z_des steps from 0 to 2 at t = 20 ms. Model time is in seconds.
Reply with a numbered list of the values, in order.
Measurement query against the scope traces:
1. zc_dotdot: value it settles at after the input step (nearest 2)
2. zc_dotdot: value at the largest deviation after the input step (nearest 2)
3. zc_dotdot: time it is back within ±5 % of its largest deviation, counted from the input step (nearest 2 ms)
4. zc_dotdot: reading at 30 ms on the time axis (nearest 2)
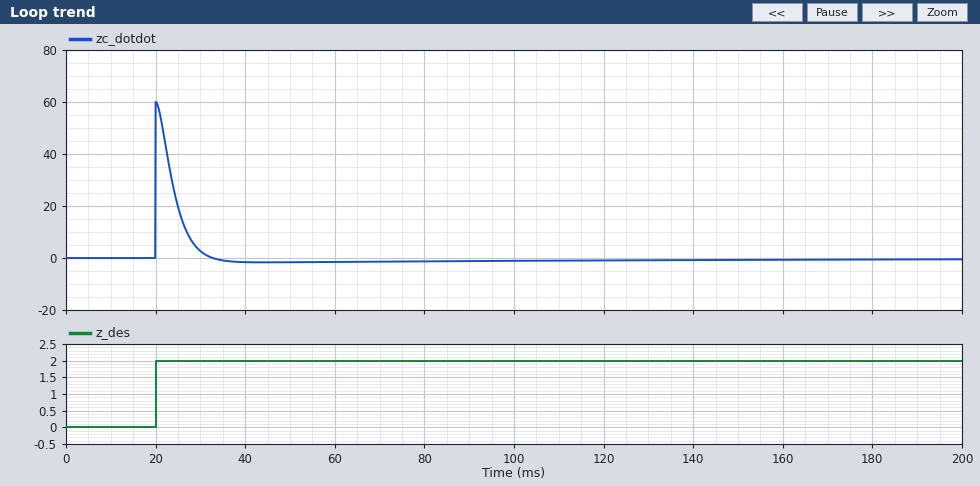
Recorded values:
1. 0
2. 60
3. 10 ms
4. 2
